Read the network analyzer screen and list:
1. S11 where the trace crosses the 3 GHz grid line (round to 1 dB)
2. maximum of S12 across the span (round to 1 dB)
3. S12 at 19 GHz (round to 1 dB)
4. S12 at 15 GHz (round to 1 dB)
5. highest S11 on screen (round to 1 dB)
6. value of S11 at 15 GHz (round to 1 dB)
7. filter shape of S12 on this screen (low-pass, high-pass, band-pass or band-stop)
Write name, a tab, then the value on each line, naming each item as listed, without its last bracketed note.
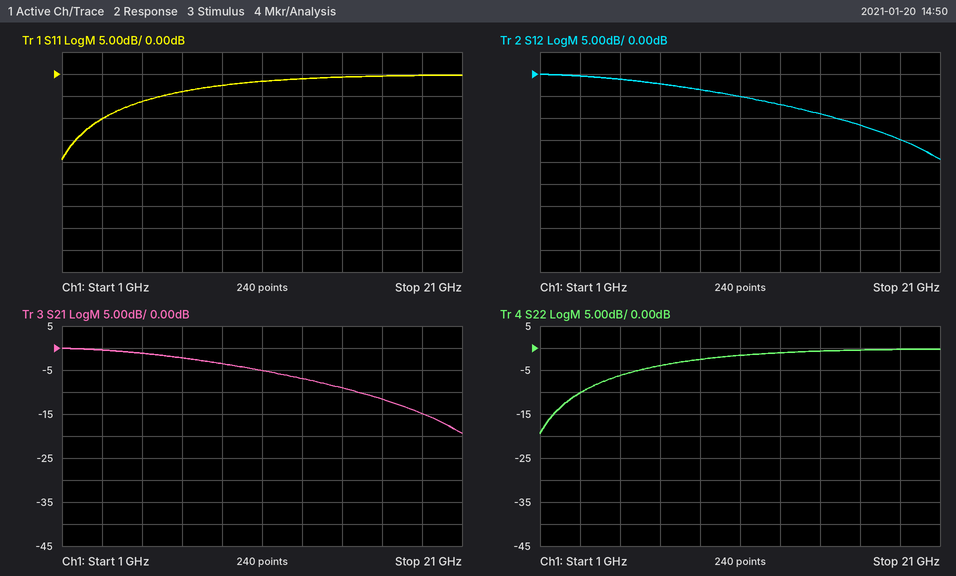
S11 where the trace crosses the 3 GHz grid line	-10 dB
maximum of S12 across the span	0 dB
S12 at 19 GHz	-15 dB
S12 at 15 GHz	-9 dB
highest S11 on screen	0 dB
value of S11 at 15 GHz	-1 dB
filter shape of S12 on this screen	low-pass
